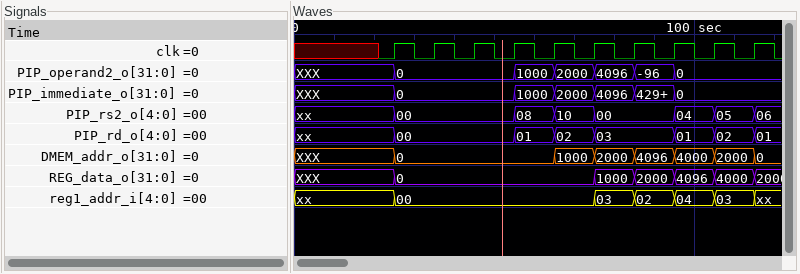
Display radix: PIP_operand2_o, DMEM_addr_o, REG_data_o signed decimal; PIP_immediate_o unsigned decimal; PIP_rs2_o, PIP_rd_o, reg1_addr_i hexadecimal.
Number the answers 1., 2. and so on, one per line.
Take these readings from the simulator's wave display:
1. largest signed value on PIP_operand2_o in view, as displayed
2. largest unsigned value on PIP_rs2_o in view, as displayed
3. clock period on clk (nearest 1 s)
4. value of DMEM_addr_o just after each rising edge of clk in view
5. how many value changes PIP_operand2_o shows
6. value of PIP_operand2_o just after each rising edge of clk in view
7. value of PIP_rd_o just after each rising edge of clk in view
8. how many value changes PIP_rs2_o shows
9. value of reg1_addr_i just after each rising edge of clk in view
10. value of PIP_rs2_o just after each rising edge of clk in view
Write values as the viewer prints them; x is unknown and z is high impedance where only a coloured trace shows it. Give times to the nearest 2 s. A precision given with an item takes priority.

1. 4096
2. 10
3. 10 s
4. 0, 0, 0, 0, 1000, 2000, 4096, 4000, 2000, 0
5. 6
6. 0, 0, 0, 1000, 2000, 4096, -96, 0, 0, 0
7. 00, 00, 00, 01, 02, 03, 03, 01, 02, 01
8. 7
9. 00, 00, 00, 00, 00, 03, 02, 04, 03, xx
10. 00, 00, 00, 08, 10, 00, 00, 04, 05, 06
